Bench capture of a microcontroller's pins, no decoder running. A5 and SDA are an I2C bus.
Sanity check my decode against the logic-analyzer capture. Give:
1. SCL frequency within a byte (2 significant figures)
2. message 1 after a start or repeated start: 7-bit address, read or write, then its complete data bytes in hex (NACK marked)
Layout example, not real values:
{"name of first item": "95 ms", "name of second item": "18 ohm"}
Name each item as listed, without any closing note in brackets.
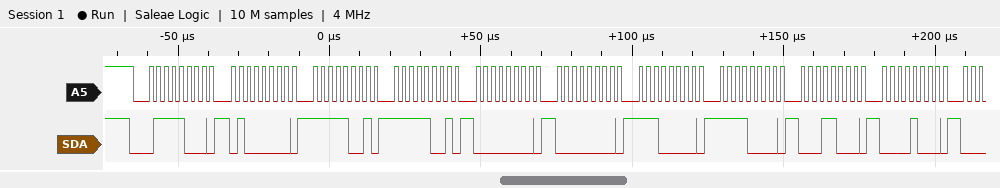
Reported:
{"SCL frequency within a byte": "400 kHz", "message 1 after a start or repeated start: 7-bit address, read or write, then its complete data bytes in hex": "0x3C write: 40 F9 F9 00 00 E0 F0 18 08"}
